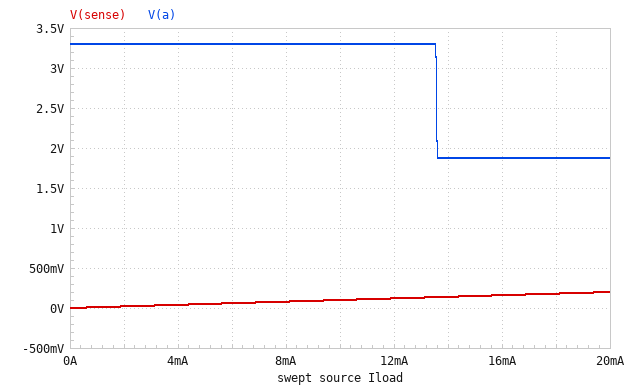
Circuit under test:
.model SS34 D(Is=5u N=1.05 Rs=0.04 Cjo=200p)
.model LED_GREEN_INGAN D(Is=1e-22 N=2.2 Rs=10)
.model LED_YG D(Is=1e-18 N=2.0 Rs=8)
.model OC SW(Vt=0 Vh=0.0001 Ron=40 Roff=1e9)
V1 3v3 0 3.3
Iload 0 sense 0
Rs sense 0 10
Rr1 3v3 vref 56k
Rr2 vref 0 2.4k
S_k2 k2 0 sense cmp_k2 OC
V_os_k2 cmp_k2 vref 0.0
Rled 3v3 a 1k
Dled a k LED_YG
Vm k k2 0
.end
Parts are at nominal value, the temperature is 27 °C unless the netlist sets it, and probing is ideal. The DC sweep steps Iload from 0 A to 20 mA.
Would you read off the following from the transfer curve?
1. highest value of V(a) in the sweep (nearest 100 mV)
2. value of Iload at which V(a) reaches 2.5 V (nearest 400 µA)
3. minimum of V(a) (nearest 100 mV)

3.3 V
13.6 mA
1.9 V
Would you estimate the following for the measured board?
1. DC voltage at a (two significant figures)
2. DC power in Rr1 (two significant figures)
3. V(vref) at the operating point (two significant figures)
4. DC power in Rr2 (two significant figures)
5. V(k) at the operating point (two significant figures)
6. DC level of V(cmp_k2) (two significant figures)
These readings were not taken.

3.3 V
180 µW
140 mV
7.7 µW
2.2 V
140 mV
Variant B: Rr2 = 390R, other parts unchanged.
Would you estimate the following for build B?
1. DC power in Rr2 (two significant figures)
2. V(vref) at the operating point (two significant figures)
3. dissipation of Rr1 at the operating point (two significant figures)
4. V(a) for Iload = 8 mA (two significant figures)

1.3 µW
23 mV
190 µW
1.9 V
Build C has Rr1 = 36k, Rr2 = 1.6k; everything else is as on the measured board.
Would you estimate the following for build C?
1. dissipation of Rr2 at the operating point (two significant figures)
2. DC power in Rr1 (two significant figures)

12 µW
280 µW
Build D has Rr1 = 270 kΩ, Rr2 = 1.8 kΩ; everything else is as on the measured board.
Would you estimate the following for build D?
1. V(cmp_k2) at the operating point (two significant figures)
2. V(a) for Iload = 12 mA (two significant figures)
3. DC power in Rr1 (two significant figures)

22 mV
1.9 V
40 µW
